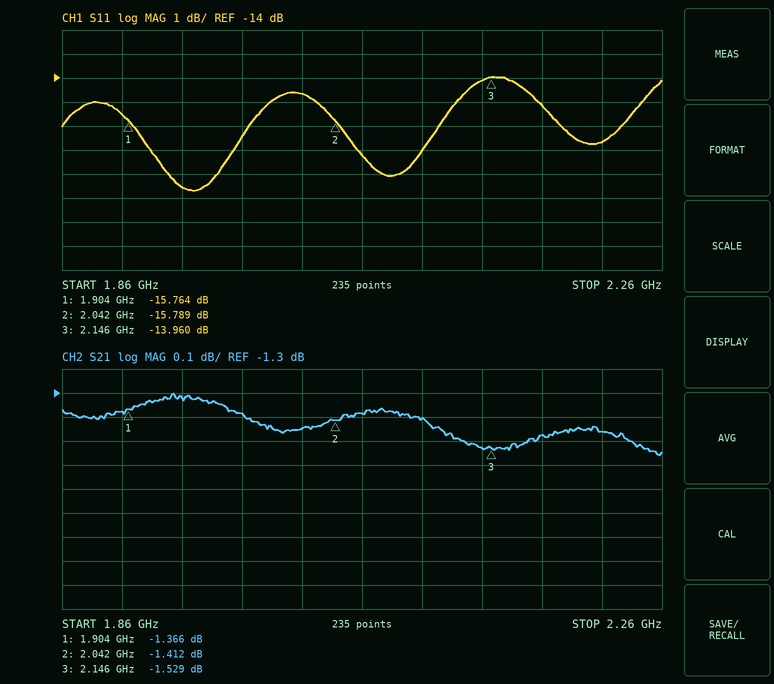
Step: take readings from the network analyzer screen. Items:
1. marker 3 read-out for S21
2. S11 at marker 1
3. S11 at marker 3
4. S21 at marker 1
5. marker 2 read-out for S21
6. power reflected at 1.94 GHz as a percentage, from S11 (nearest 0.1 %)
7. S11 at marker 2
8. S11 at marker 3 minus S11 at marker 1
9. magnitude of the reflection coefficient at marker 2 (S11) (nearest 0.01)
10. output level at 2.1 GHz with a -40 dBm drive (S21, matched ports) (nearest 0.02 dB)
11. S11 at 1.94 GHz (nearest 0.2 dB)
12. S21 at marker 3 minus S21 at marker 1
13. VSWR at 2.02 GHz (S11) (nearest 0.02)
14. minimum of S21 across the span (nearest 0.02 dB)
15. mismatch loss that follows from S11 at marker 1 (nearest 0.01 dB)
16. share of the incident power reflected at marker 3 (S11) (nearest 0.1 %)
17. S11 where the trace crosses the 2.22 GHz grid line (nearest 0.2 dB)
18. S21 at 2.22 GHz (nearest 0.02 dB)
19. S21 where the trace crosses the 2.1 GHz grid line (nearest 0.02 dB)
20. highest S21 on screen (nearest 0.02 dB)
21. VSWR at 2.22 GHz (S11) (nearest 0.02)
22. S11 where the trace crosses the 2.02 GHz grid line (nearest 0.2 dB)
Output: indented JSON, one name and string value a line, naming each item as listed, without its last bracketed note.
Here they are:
{
  "marker 3 read-out for S21": "-1.529 dB",
  "S11 at marker 1": "-15.764 dB",
  "S11 at marker 3": "-13.960 dB",
  "S21 at marker 1": "-1.366 dB",
  "marker 2 read-out for S21": "-1.412 dB",
  "power reflected at 1.94 GHz as a percentage, from S11": "1.4 %",
  "S11 at marker 2": "-15.789 dB",
  "S11 at marker 3 minus S11 at marker 1": "1.804 dB",
  "magnitude of the reflection coefficient at marker 2 (S11)": "0.16",
  "output level at 2.1 GHz with a -40 dBm drive (S21, matched ports)": "-41.40 dBm",
  "S11 at 1.94 GHz": "-18.6 dB",
  "S21 at marker 3 minus S21 at marker 1": "-0.163 dB",
  "VSWR at 2.02 GHz (S11)": "1.46",
  "minimum of S21 across the span": "-1.56 dB",
  "mismatch loss that follows from S11 at marker 1": "0.12 dB",
  "share of the incident power reflected at marker 3 (S11)": "4.0 %",
  "S11 where the trace crosses the 2.22 GHz grid line": "-16.6 dB",
  "S21 at 2.22 GHz": "-1.46 dB",
  "S21 where the trace crosses the 2.1 GHz grid line": "-1.40 dB",
  "highest S21 on screen": "-1.30 dB",
  "VSWR at 2.22 GHz (S11)": "1.34",
  "S11 where the trace crosses the 2.02 GHz grid line": "-14.6 dB"
}
